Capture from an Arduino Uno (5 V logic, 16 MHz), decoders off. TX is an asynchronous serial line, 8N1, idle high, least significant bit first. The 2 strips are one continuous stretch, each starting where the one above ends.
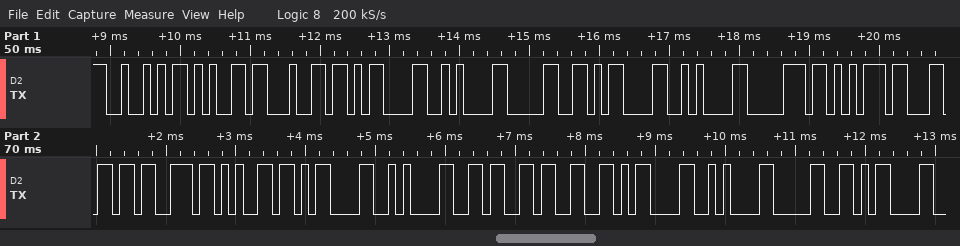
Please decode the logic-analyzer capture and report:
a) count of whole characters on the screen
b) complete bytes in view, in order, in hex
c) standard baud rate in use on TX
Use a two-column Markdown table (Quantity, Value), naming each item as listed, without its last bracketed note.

| Quantity | Value |
|---|---|
| count of whole characters on the screen | 21 |
| complete bytes in view, in order, in hex | 52 65 64 0D 0A 30 0D 0A 70 75 6C 73 65 0D 0A 36 33 0D 0A 30 0D |
| standard baud rate in use on TX | 9600 baud |
